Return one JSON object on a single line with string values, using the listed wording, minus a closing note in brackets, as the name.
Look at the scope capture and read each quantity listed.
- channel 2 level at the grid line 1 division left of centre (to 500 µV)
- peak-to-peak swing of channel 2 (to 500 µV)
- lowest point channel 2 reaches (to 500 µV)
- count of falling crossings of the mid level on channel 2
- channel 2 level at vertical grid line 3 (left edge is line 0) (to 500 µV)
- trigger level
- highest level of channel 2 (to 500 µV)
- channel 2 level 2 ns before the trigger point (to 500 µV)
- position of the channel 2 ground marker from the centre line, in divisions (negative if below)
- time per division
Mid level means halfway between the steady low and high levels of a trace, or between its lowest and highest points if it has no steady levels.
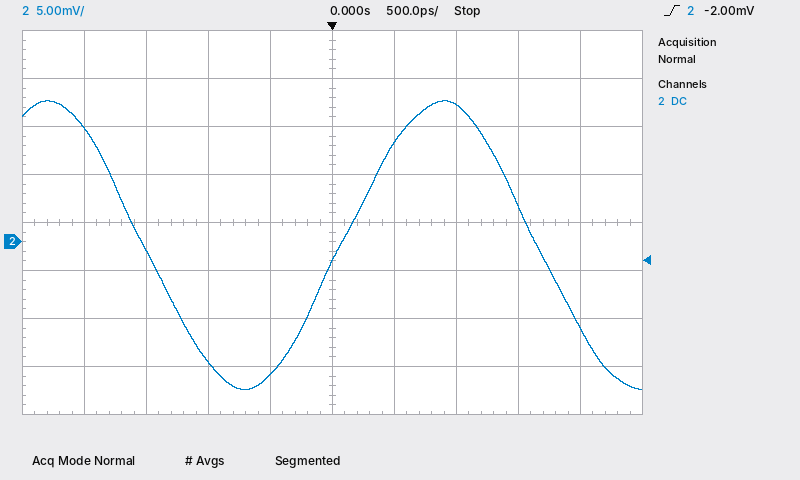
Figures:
{"channel 2 level at the grid line 1 division left of centre": "-14.0 mV", "peak-to-peak swing of channel 2": "30.0 mV", "lowest point channel 2 reaches": "-15.5 mV", "count of falling crossings of the mid level on channel 2": "2", "channel 2 level at vertical grid line 3 (left edge is line 0)": "-12.5 mV", "trigger level": "-2.00 mV", "highest level of channel 2": "14.5 mV", "channel 2 level 2 ns before the trigger point": "12.0 mV", "position of the channel 2 ground marker from the centre line, in divisions": "-0.4 div", "time per division": "500 ps"}
